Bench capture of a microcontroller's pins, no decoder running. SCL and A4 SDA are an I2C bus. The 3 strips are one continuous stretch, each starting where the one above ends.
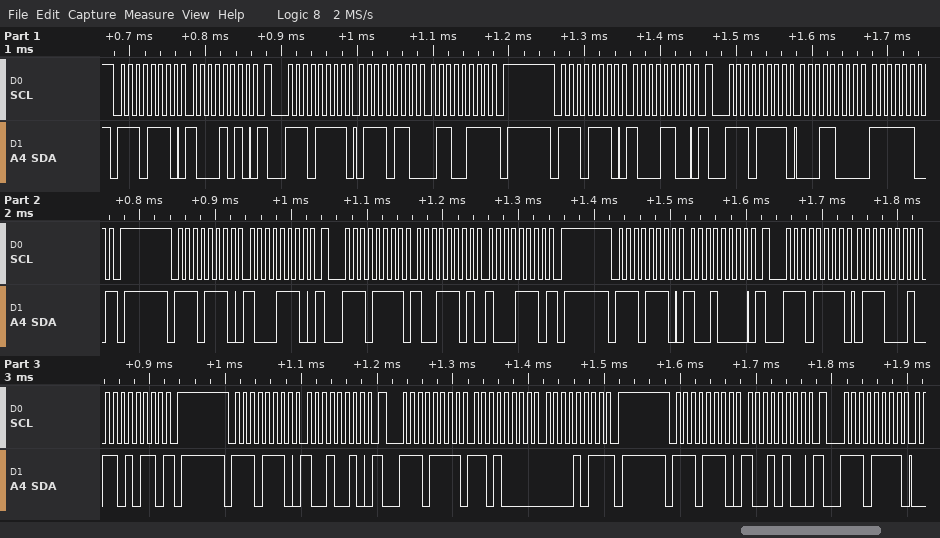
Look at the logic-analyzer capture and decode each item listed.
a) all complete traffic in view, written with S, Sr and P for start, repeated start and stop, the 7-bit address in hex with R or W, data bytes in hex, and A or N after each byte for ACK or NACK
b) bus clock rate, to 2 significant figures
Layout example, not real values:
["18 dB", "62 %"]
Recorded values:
["S 77W A 8A A Sr 77R A 76 A 67 N P S 77W A 8C A Sr 77R A 18 A FC N P S 77W A 8E A Sr 77R A 9D A 8E N P S 77W A 90 A Sr 77R A 71 A D6 N P S 77W A 92 A Sr 77R A D0 A 0B N P S 77W A 94 A Sr 77R A", "100 kHz"]
